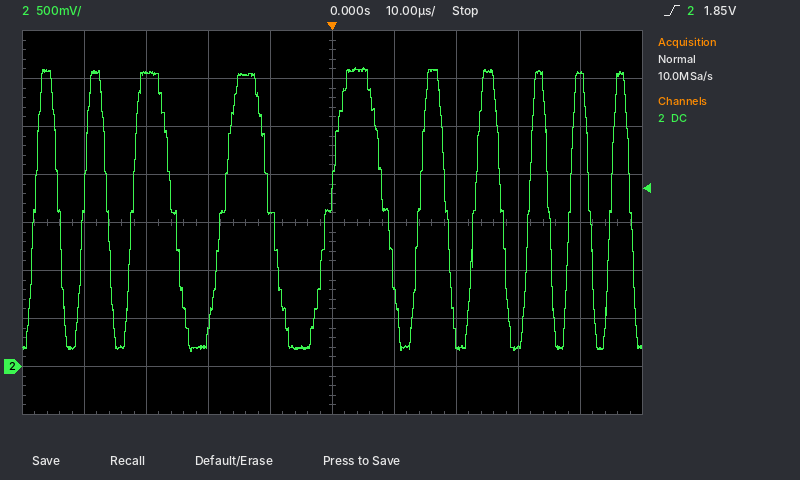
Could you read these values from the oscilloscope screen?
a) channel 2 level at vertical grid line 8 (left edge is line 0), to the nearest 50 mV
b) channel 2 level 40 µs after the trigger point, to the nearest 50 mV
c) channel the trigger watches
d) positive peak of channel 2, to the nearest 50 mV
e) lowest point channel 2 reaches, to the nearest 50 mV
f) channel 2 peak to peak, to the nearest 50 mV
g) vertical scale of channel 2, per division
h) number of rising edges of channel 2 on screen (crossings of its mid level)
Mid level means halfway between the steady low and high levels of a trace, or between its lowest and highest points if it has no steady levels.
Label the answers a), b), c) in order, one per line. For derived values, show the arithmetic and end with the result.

a) 200 mV
b) 3.05 V
c) channel 2
d) 3.10 V
e) 150 mV
f) 3.10 V − (150 mV) = 2.95 V
g) 500 mV
h) 10
